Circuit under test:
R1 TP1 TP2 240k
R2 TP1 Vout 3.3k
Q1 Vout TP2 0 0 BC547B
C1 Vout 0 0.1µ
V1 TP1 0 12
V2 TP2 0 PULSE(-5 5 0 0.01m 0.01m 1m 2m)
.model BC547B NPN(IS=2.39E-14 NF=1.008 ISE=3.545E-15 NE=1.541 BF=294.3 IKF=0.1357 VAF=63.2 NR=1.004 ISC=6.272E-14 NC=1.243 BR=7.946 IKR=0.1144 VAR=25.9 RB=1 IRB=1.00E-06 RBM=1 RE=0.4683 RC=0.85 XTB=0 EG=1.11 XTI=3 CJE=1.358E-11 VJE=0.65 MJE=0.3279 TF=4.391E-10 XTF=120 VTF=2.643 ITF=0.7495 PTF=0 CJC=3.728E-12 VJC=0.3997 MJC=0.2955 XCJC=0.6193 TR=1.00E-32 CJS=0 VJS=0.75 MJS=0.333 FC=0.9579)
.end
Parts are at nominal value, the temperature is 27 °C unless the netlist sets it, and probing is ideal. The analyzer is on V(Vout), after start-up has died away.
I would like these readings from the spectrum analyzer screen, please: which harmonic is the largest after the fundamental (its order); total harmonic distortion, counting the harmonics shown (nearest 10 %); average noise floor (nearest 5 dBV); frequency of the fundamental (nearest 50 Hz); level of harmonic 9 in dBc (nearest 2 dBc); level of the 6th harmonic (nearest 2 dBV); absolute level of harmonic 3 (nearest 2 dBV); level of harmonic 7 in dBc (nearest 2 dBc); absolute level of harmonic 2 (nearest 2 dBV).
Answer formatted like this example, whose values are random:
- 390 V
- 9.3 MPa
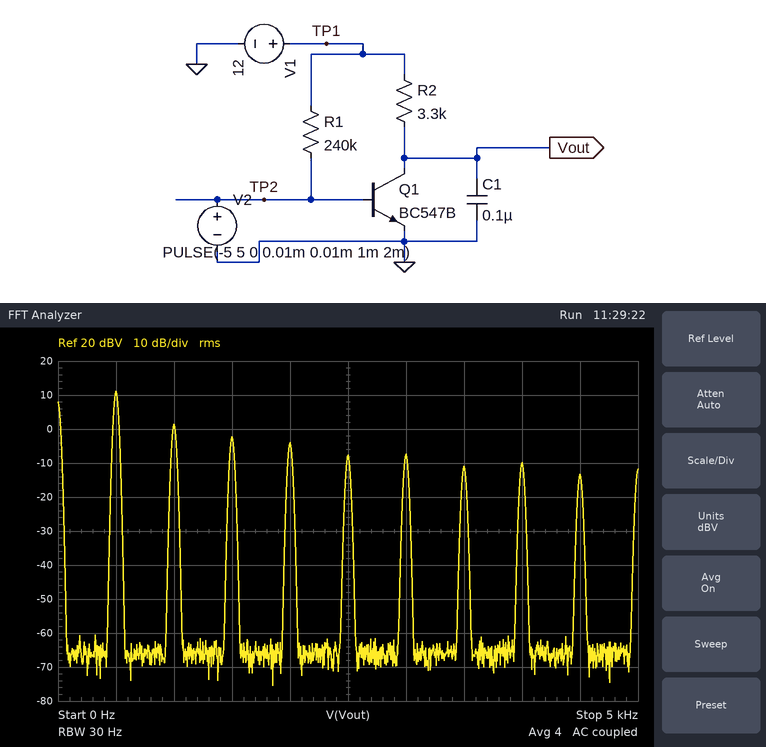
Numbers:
- 2
- 50 %
- -65 dBV
- 500 Hz
- -24 dBc
- -8 dBV
- -2 dBV
- -22 dBc
- 2 dBV
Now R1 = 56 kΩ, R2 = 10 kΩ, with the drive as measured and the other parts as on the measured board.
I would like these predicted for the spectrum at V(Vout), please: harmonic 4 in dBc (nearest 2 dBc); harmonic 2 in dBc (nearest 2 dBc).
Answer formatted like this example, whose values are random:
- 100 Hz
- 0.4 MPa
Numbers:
- -12 dBc
- -6 dBc
